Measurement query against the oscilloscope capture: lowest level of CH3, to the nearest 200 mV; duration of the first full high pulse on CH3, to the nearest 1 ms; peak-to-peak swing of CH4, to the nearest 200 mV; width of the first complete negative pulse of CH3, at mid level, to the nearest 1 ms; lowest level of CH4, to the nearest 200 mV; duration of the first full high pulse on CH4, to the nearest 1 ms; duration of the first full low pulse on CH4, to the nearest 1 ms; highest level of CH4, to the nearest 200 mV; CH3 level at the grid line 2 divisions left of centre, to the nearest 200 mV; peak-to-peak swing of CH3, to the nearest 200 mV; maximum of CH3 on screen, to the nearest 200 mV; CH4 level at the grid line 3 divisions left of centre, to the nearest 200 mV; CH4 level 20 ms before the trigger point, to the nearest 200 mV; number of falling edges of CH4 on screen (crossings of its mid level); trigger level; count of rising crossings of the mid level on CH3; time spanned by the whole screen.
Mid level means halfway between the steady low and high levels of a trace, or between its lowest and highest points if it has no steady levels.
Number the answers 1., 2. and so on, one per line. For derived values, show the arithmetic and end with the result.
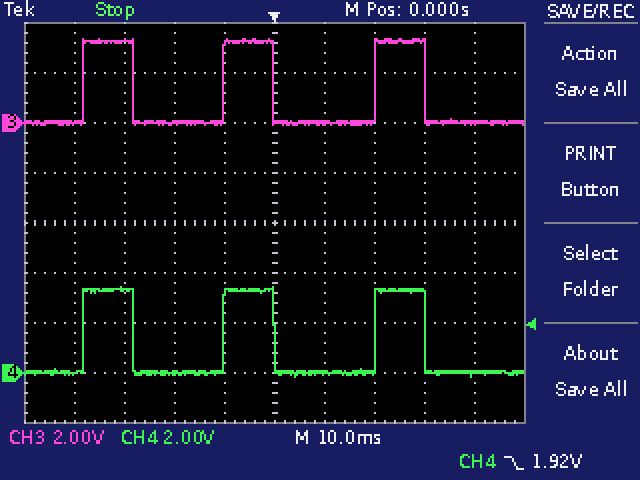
1. 0.0 V
2. 10 ms
3. 3.4 V − (-200 mV) = 3.6 V
4. 18 ms
5. -200 mV
6. 10 ms
7. 18 ms
8. 3.4 V
9. 0.0 V
10. 3.4 V − (0.0 V) = 3.4 V
11. 3.4 V
12. 3.4 V
13. 0.0 V
14. 3
15. 1.92 V
16. 3
17. 100 ms
